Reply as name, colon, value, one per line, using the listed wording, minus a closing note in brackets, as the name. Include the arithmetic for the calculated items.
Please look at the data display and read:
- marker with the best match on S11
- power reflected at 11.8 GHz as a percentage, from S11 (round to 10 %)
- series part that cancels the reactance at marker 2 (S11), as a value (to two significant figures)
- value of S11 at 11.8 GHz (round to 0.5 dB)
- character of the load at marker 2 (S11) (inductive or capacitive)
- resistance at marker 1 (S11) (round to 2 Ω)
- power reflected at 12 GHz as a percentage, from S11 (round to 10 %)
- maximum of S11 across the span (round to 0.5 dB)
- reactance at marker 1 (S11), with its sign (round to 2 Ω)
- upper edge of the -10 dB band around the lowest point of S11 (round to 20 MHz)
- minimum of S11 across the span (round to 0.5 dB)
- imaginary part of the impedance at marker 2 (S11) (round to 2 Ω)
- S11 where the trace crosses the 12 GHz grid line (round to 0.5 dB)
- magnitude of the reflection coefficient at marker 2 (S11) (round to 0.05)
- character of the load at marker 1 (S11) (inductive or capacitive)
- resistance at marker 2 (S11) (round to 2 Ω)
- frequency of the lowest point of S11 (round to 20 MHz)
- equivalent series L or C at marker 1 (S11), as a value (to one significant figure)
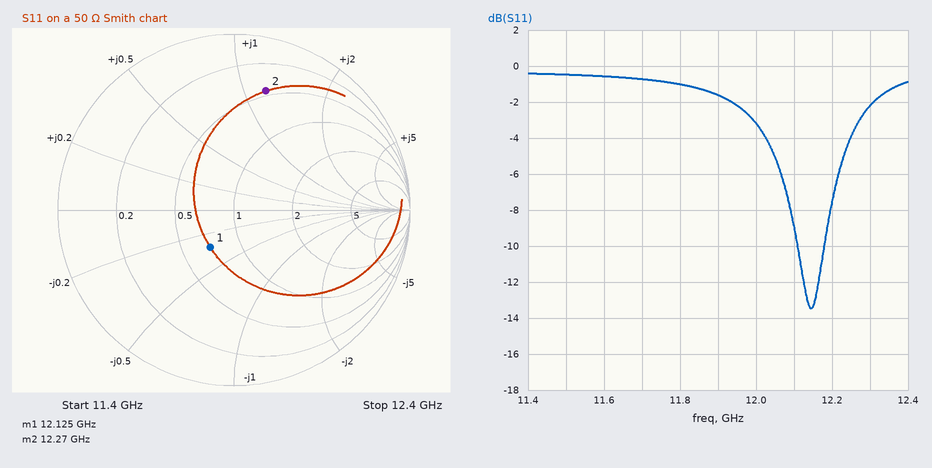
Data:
marker with the best match on S11: marker 1
power reflected at 11.8 GHz as a percentage, from S11: 10^(-1/10) ≈ 79.4 %, so 80 % to the nearest 10 %
series part that cancels the reactance at marker 2 (S11), as a value: C = 1/(2π × 12.27 GHz × 60 Ω) ≈ 216 fF, so 220 fF to two significant figures
value of S11 at 11.8 GHz: -1.0 dB
character of the load at marker 2 (S11): inductive
resistance at marker 1 (S11): 36 Ω
power reflected at 12 GHz as a percentage, from S11: 10^(-3/10) ≈ 50 %
maximum of S11 across the span: -0.5 dB
reactance at marker 1 (S11), with its sign: -16 Ω
upper edge of the -10 dB band around the lowest point of S11: 12.18 GHz
minimum of S11 across the span: -13.5 dB
imaginary part of the impedance at marker 2 (S11): +60 Ω
S11 where the trace crosses the 12 GHz grid line: -3.0 dB
magnitude of the reflection coefficient at marker 2 (S11): 0.70
character of the load at marker 1 (S11): capacitive
resistance at marker 2 (S11): 22 Ω
frequency of the lowest point of S11: 12.14 GHz
equivalent series L or C at marker 1 (S11), as a value: C = 1/(2π × 12.125 GHz × 16 Ω) ≈ 820 fF, so 800 fF to one significant figure
